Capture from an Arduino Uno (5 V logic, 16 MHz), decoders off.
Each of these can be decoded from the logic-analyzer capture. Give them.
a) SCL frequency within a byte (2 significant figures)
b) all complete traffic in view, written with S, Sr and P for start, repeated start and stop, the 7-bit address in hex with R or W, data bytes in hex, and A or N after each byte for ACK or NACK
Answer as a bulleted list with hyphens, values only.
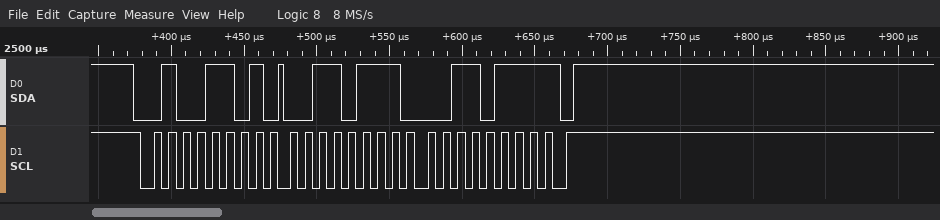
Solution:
- 100 kHz
- S 26R A 37 A 37 N P
